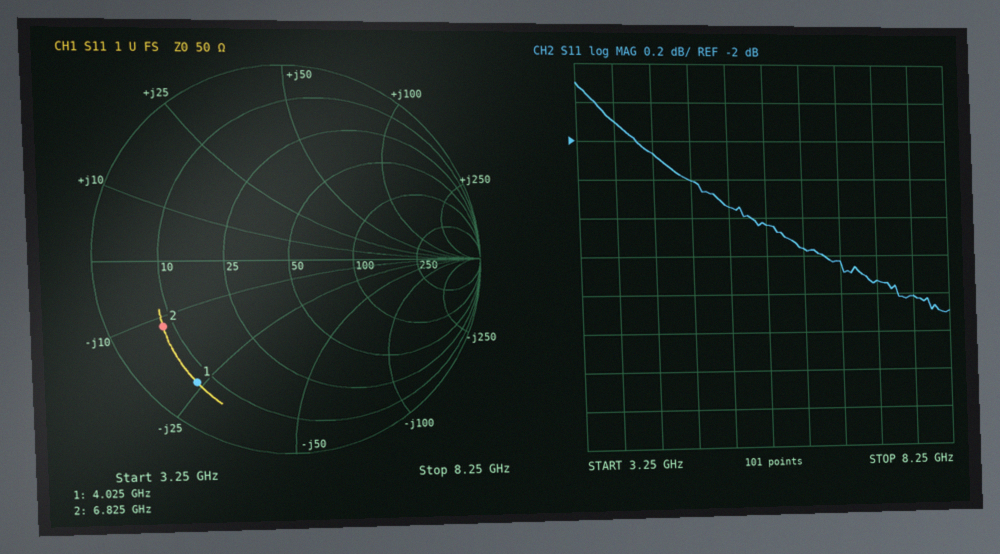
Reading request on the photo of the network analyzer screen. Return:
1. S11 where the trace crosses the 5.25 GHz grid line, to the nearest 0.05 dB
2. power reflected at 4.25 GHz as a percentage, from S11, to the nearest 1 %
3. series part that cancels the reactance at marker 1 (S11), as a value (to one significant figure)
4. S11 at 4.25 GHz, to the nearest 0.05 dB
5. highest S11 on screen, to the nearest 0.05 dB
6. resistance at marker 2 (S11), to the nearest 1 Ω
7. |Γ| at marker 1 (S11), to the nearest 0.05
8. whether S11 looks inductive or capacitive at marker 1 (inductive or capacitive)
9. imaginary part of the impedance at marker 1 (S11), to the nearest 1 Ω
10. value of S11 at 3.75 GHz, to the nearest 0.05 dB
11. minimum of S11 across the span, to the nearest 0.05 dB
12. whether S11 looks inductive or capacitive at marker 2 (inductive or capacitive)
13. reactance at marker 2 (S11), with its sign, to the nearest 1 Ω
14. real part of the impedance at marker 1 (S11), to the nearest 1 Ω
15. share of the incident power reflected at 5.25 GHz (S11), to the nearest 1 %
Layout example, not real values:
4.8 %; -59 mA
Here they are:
-2.35 dB; 62 %; 900 pH; -2.05 dB; -1.70 dB; 8 Ω; 0.80; capacitive; -24 Ω; -1.90 dB; -2.90 dB; capacitive; -12 Ω; 7 Ω; 58 %
